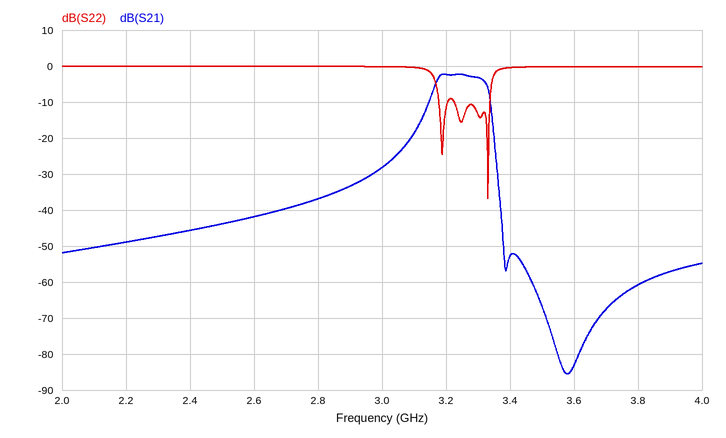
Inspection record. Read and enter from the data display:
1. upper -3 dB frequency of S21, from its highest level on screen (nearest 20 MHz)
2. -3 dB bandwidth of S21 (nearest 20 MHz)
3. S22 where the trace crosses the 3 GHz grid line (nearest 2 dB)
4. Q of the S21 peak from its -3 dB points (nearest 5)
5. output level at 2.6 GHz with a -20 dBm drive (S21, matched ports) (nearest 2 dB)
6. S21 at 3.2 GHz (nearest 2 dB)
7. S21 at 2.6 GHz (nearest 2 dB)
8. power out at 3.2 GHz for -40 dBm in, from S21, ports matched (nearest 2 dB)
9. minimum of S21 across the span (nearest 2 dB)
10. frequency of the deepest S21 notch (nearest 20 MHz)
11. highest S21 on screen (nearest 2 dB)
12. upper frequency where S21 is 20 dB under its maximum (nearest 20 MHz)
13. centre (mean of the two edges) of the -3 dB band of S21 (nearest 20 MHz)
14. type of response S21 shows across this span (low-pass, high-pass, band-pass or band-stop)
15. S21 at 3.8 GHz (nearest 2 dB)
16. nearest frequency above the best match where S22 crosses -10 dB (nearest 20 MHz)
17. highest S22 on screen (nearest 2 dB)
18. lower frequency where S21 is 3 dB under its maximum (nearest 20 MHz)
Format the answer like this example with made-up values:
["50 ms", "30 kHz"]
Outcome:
["3.32 GHz", "160 MHz", "0 dB", "20", "-62 dBm", "-2 dB", "-42 dB", "-42 dBm", "-86 dB", "3.58 GHz", "-2 dB", "3.36 GHz", "3.24 GHz", "band-pass", "-60 dB", "3.34 GHz", "0 dB", "3.16 GHz"]
